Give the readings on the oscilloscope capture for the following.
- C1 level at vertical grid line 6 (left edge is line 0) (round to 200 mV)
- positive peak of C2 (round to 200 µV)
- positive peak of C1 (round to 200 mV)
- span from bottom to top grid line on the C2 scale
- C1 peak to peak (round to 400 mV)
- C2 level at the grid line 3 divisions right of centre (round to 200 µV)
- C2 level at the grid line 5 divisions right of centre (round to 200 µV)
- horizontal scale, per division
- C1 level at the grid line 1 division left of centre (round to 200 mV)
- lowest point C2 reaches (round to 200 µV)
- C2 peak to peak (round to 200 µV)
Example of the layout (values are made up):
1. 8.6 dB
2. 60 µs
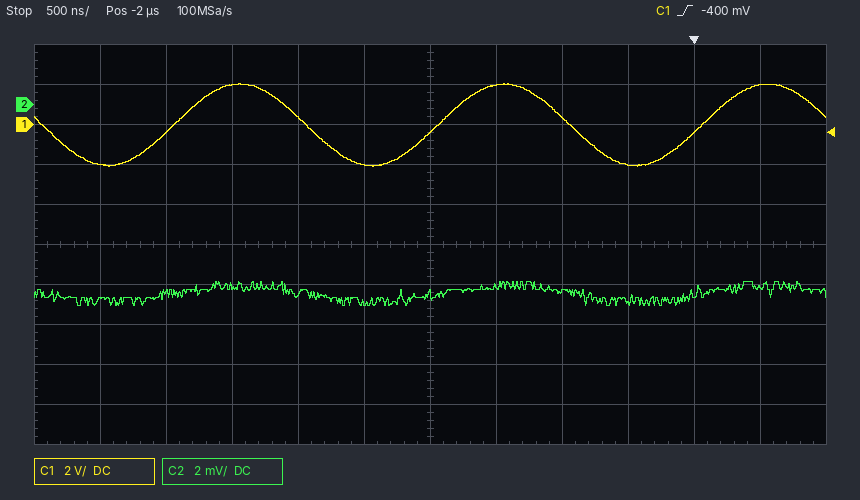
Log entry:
1. -400 mV
2. -8.8 mV
3. 2.0 V
4. 20 mV
5. 4.0 V
6. -9.8 mV
7. -9.2 mV
8. 500 ns
9. -2.0 V
10. -10.0 mV
11. 1.2 mV
